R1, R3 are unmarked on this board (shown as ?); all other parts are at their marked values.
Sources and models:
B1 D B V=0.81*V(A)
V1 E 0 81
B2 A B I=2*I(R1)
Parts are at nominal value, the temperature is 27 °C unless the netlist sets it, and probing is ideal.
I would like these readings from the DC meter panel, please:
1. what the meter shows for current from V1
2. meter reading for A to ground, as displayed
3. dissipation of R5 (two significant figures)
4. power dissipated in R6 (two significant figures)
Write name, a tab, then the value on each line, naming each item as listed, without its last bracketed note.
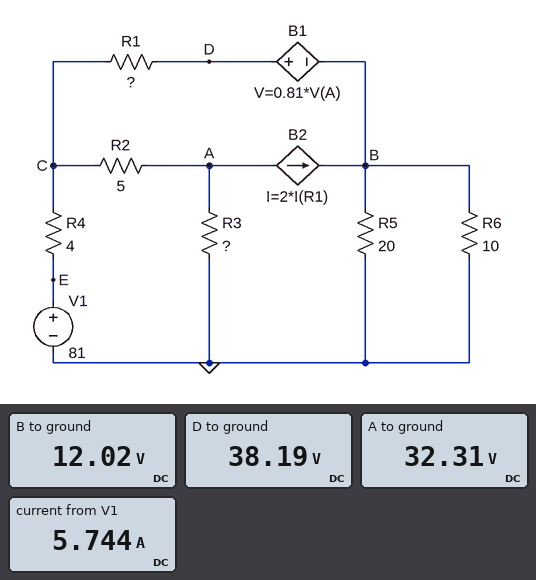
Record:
what the meter shows for current from V1	5.744 A
meter reading for A to ground, as displayed	32.31 V
dissipation of R5	7.2 W
power dissipated in R6	14 W
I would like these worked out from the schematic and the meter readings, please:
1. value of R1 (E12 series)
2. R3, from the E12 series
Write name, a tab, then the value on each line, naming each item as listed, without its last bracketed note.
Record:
value of R1	33 Ω
R3, from the E12 series	8.2 Ω
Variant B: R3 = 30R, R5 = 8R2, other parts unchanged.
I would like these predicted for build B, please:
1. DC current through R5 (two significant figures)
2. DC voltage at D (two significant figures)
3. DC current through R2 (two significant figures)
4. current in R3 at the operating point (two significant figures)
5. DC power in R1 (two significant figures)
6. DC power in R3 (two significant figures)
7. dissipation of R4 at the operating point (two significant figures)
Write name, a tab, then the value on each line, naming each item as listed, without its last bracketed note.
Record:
DC current through R5	860 mA
DC voltage at D	50 V
DC current through R2	2.8 A
current in R3 at the operating point	1.8 A
DC power in R1	9.0 W
DC power in R3	95 W
dissipation of R4 at the operating point	45 W
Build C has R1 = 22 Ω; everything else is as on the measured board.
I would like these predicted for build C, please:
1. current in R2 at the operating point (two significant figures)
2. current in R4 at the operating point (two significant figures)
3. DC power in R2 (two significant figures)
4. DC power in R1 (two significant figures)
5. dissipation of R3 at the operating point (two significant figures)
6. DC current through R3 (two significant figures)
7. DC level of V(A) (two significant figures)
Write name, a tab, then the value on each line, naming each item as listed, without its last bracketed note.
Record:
current in R2 at the operating point	5.3 A
current in R4 at the operating point	6.0 A
DC power in R2	140 W
DC power in R1	13 W
dissipation of R3 at the operating point	110 W
DC current through R3	3.7 A
DC level of V(A)	31 V
